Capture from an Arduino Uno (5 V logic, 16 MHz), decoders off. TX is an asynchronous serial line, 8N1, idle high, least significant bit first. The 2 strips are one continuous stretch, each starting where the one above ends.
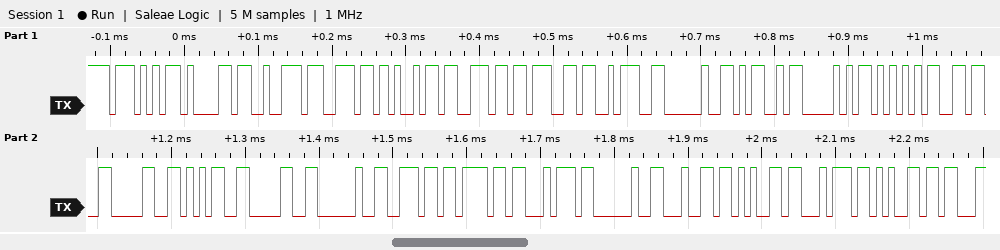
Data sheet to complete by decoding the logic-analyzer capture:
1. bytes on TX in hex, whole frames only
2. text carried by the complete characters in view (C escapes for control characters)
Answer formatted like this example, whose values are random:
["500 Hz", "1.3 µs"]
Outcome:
["0x57 0x61 0x72 0x6E 0x69 0x6E 0x67 0x3A 0x20 0x4D 0x50 0x55 0x36 0x30 0x35 0x30 0x20 0x6E 0x6F 0x74 0x20 0x64 0x65 0x74 0x65", "\"Warning: MPU6050 not dete\""]
